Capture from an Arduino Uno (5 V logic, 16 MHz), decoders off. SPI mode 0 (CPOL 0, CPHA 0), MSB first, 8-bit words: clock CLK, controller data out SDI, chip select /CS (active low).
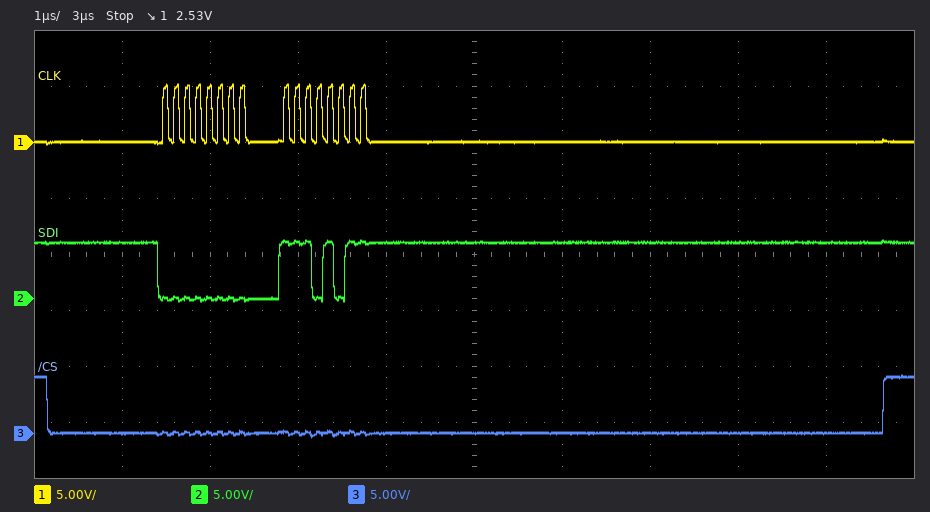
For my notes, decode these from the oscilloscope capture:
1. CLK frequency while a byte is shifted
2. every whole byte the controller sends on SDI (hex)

8 MHz
00 EB
